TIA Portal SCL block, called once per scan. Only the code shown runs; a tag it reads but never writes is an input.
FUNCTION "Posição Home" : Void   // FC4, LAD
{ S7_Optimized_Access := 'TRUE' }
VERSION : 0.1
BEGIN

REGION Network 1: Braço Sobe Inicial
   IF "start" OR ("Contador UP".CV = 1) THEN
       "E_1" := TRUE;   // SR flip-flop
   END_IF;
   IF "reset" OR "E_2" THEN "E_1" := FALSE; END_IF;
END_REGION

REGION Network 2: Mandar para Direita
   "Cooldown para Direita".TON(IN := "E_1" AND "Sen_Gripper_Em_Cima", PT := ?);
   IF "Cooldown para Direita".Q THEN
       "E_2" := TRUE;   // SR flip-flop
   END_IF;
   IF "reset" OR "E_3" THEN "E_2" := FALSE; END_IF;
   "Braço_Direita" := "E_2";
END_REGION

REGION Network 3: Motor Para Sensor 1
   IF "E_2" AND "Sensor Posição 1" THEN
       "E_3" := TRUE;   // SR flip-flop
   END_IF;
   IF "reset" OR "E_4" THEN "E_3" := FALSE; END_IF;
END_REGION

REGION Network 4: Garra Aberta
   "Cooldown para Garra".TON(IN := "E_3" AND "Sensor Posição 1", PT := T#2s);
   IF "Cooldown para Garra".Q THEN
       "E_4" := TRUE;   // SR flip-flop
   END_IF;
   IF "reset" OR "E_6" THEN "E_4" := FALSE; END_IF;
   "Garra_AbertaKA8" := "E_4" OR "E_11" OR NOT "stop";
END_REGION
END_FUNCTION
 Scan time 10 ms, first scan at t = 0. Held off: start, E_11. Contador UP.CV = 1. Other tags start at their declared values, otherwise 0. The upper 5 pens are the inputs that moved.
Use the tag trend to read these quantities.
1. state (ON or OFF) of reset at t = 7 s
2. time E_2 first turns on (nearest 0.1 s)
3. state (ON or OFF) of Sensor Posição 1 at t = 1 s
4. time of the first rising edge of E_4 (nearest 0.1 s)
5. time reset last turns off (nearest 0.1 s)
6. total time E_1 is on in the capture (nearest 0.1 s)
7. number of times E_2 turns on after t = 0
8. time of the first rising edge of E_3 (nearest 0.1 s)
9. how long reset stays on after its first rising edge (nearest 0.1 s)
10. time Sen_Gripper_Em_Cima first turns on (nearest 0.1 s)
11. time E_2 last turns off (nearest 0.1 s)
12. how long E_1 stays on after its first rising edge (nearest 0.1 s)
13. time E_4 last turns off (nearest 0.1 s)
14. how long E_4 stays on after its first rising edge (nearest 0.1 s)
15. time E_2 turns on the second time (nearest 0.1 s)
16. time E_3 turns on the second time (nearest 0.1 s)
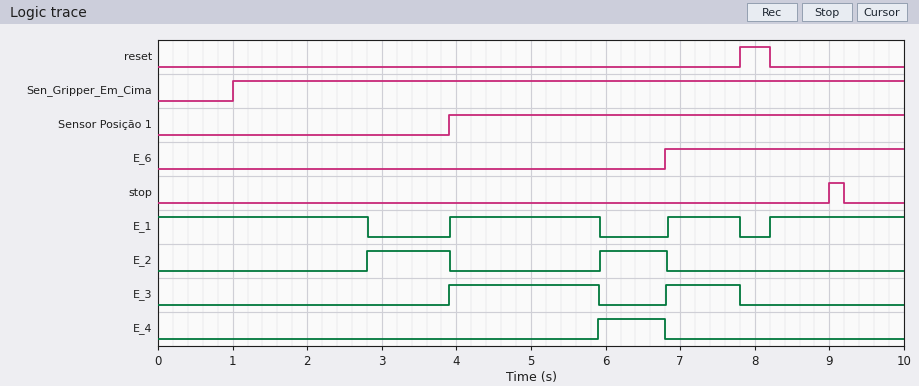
OFF
2.8 s
OFF
5.9 s
8.2 s
7.6 s
2
3.9 s
0.4 s
1.0 s
6.8 s
2.0 s
6.8 s
0.9 s
5.9 s
6.8 s
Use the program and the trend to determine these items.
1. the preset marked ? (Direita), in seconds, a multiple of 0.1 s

1.8 s
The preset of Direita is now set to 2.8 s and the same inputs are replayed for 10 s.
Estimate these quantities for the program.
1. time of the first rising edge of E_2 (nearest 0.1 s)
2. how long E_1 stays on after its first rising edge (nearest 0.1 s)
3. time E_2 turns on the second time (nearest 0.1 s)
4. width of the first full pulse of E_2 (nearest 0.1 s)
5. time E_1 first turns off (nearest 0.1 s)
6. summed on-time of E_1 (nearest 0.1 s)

3.8 s
2.8 s
6.7 s
0.1 s
3.8 s
9.4 s
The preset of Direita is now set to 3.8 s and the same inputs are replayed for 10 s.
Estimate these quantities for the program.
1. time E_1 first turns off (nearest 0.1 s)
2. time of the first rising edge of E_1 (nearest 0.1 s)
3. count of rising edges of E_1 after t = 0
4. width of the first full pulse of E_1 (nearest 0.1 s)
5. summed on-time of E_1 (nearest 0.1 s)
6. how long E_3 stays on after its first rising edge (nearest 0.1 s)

4.8 s
4.8 s
2
3.0 s
9.6 s
3.0 s
